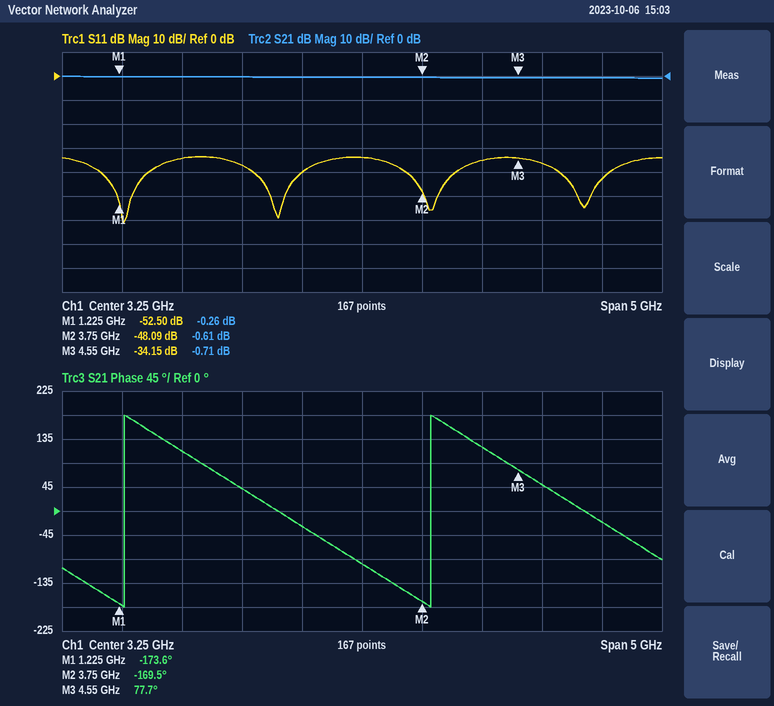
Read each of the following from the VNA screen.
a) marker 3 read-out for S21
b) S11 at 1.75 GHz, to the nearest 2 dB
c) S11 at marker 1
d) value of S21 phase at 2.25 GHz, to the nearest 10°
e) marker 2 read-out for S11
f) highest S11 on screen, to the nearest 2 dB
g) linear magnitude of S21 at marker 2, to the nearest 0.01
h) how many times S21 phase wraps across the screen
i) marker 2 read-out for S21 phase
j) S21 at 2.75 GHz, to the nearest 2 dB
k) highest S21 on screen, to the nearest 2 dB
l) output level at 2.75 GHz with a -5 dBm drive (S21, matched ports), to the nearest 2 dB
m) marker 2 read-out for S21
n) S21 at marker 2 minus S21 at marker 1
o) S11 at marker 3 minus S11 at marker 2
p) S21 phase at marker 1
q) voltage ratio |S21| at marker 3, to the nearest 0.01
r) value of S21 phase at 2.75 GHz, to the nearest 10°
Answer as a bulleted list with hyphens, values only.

- -0.71 dB
- -34 dB
- -52.50 dB
- 40°
- -48.09 dB
- -34 dB
- 0.93
- 2
- -169.5°
- 0 dB
- 0 dB
- -6 dBm
- -0.61 dB
- -0.35 dB
- 13.94 dB
- -173.6°
- 0.92
- -30°
